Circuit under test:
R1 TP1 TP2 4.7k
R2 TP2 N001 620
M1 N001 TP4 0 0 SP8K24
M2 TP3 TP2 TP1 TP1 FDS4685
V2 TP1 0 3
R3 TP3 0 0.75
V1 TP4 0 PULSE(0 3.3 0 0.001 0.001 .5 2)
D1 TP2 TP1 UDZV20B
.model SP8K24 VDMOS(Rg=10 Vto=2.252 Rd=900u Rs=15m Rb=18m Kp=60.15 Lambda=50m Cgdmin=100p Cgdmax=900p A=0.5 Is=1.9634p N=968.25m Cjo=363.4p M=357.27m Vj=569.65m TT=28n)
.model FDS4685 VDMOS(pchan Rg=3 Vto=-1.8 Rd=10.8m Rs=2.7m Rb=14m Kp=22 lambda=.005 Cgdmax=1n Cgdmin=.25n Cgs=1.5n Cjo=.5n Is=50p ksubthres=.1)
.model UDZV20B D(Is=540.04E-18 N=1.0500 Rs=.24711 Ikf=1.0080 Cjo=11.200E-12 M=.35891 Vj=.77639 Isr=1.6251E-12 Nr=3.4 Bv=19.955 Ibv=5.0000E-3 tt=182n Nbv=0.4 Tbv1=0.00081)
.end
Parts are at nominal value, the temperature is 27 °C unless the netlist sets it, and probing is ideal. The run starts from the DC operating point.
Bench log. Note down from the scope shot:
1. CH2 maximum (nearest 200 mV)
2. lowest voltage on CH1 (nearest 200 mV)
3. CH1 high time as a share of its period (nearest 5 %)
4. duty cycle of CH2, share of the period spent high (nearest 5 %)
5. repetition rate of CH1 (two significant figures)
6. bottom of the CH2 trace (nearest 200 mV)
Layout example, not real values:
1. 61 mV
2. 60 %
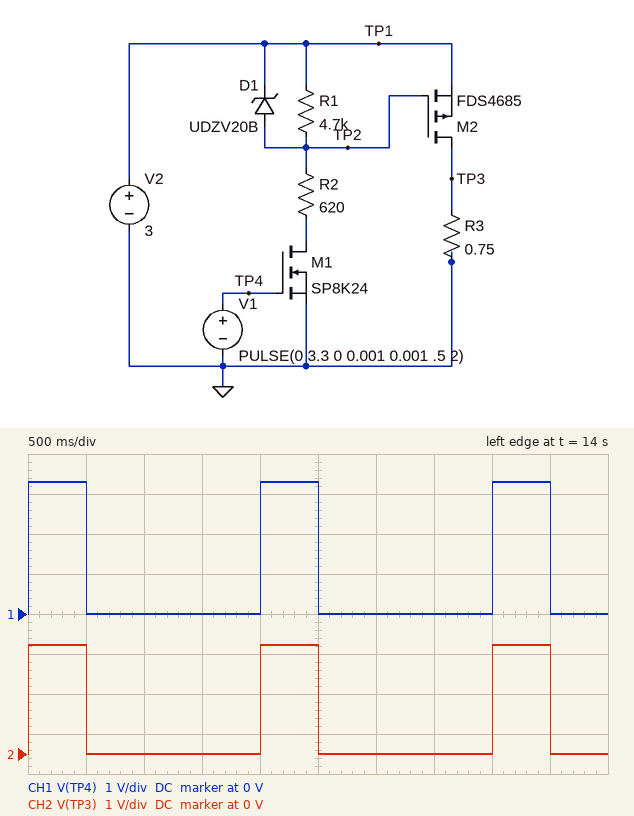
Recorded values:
1. 2.8 V
2. 0 V
3. 25 %
4. 25 %
5. 500 mHz
6. 0 V
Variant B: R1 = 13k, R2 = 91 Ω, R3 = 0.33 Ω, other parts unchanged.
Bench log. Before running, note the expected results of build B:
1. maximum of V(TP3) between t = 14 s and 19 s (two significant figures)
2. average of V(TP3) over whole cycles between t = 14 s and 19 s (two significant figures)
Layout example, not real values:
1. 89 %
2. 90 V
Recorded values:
1. 2.5 V
2. 640 mV
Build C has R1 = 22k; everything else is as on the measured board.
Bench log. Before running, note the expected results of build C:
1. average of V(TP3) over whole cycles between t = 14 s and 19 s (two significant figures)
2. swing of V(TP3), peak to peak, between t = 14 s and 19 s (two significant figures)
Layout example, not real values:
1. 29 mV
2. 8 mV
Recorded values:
1. 700 mV
2. 2.8 V
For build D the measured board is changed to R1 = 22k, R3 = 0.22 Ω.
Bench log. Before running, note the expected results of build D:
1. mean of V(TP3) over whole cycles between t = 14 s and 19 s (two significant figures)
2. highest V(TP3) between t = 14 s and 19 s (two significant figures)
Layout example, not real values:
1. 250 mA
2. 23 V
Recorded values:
1. 570 mV
2. 2.3 V
